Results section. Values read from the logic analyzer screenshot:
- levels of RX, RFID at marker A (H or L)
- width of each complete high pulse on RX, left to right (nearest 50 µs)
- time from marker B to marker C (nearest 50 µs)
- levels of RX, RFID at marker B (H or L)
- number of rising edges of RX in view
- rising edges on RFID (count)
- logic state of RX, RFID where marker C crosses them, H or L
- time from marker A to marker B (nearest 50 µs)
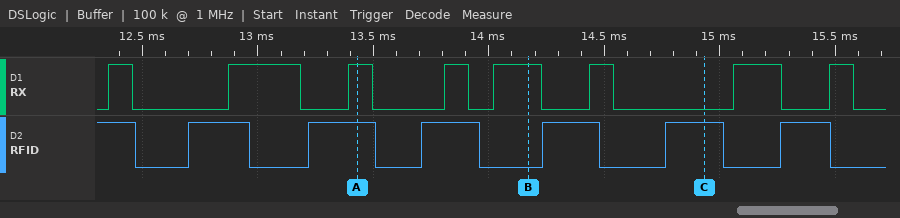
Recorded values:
RX=H, RFID=H
100 µs, 300 µs, 100 µs, 100 µs, 200 µs, 100 µs, 200 µs, 100 µs
750 µs
RX=H, RFID=L
8
6
RX=L, RFID=H
750 µs
